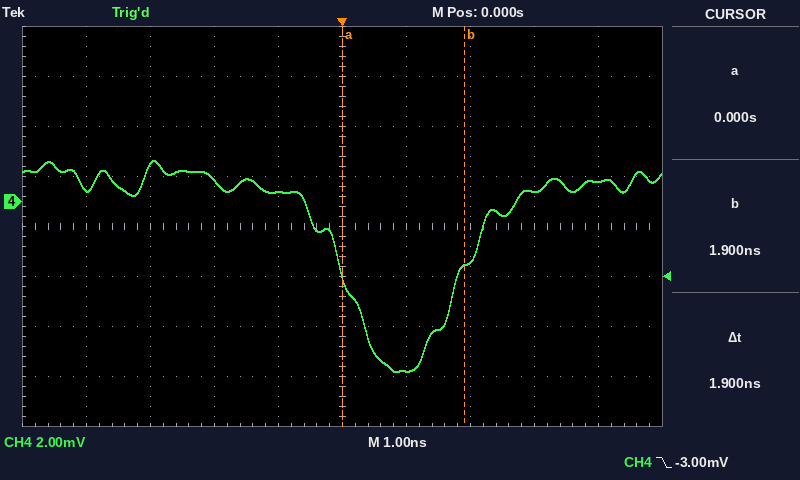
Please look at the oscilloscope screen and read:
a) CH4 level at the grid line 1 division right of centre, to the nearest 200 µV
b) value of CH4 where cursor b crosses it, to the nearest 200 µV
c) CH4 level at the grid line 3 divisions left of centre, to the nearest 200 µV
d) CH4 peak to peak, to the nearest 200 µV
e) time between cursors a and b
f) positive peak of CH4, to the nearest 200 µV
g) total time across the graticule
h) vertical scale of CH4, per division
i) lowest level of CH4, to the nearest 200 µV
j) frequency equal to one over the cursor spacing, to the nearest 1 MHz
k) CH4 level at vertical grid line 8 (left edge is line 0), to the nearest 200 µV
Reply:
-6.8 mV
-2.6 mV
1.4 mV
8.4 mV
1.9 ns
1.6 mV
10 ns
2 mV
-6.8 mV
526 MHz
400 µV
